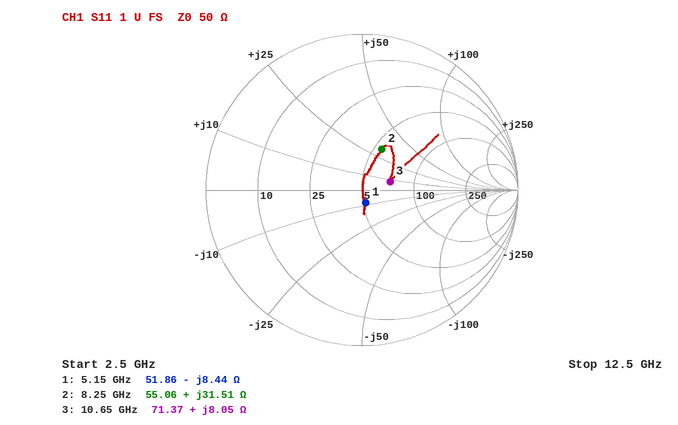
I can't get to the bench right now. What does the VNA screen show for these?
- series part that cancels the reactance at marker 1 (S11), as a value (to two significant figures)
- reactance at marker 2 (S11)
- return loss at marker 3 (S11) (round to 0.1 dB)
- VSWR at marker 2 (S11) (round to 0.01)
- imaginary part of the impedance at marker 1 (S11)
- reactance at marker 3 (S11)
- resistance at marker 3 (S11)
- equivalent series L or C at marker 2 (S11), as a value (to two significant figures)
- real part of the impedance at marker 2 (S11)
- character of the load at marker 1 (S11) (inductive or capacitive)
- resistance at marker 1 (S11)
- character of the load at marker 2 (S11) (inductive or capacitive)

260 pH
+31.51 Ω
14.5 dB
1.82
-8.44 Ω
+8.05 Ω
71.37 Ω
610 pH
55.06 Ω
capacitive
51.86 Ω
inductive
